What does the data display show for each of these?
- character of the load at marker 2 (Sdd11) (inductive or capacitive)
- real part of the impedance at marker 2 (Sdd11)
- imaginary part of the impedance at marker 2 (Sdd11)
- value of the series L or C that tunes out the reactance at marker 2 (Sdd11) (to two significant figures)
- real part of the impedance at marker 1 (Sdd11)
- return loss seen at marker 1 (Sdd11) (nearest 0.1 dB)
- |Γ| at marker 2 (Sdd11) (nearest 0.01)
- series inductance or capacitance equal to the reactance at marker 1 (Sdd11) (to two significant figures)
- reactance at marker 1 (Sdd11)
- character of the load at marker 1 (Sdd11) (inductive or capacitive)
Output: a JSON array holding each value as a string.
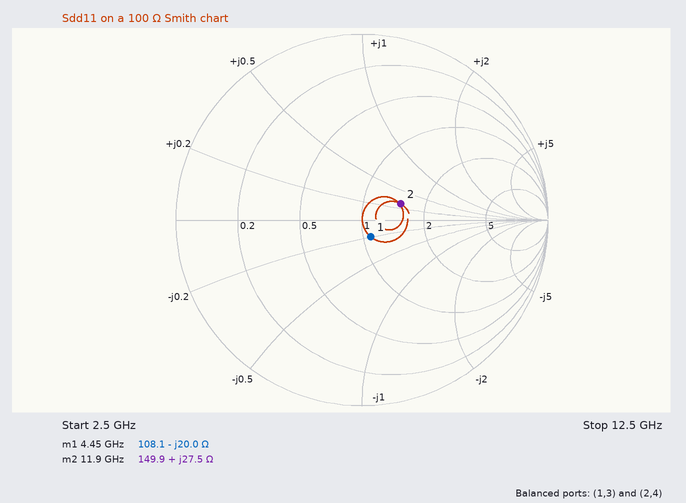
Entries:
["inductive", "149.9 Ω", "+27.5 Ω", "490 fF", "108.1 Ω", "19.7 dB", "0.23", "1.8 pF", "-20.0 Ω", "capacitive"]
